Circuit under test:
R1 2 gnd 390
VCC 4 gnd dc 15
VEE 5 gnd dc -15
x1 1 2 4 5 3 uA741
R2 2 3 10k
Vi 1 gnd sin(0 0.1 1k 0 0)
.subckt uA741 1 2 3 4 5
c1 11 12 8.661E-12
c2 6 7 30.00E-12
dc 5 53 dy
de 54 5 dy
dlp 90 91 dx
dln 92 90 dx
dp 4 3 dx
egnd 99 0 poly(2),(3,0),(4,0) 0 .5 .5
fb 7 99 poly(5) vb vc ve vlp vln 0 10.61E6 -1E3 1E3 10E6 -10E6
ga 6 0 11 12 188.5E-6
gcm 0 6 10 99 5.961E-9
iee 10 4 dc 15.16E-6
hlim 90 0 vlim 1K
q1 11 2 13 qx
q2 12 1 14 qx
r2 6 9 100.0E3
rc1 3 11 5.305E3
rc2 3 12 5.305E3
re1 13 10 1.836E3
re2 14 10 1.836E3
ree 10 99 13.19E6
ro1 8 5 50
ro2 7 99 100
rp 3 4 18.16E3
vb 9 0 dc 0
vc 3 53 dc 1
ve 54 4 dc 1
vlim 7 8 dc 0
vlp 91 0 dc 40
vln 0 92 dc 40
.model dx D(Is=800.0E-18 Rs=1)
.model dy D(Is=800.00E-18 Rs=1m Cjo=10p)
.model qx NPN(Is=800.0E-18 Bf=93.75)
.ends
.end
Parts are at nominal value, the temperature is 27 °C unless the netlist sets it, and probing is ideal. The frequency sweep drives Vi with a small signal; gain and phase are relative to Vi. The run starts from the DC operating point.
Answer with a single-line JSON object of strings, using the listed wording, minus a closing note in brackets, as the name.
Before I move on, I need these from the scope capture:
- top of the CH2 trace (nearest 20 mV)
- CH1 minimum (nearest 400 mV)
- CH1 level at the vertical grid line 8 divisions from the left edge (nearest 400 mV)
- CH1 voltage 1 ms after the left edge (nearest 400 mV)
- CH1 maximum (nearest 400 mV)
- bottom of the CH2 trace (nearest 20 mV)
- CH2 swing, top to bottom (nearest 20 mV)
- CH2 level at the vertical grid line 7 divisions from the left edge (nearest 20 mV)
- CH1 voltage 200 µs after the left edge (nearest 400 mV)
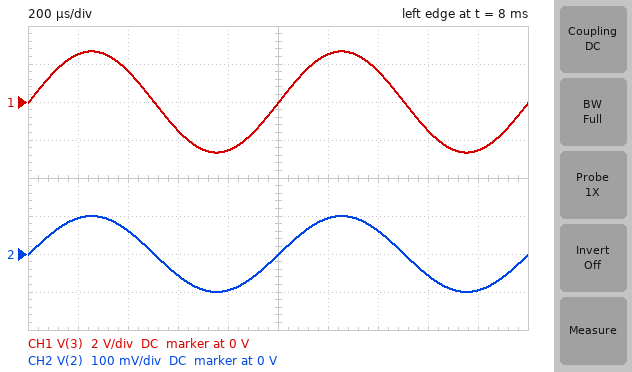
{"top of the CH2 trace": "100 mV", "CH1 minimum": "-2.8 V", "CH1 level at the vertical grid line 8 divisions from the left edge": "-1.6 V", "CH1 voltage 1 ms after the left edge": "0 V", "CH1 maximum": "2.8 V", "bottom of the CH2 trace": "-100 mV", "CH2 swing, top to bottom": "200 mV", "CH2 level at the vertical grid line 7 divisions from the left edge": "60 mV", "CH1 voltage 200 µs after the left edge": "2.4 V"}
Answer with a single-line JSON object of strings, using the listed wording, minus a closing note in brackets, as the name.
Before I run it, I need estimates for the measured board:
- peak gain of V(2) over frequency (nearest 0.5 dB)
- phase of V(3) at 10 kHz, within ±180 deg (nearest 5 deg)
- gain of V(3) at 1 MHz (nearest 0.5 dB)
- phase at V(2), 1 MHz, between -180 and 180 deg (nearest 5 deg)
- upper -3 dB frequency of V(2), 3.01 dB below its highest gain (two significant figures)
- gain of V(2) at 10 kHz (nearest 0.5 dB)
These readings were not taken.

{"peak gain of V(2) over frequency": "0 dB", "phase of V(3) at 10 kHz, within ±180 deg": "-15 deg", "gain of V(3) at 1 MHz": "-1.0 dB", "phase at V(2), 1 MHz, between -180 and 180 deg": "-120 deg", "upper -3 dB frequency of V(2), 3.01 dB below its highest gain": "38 kHz", "gain of V(2) at 10 kHz": "-0.5 dB"}
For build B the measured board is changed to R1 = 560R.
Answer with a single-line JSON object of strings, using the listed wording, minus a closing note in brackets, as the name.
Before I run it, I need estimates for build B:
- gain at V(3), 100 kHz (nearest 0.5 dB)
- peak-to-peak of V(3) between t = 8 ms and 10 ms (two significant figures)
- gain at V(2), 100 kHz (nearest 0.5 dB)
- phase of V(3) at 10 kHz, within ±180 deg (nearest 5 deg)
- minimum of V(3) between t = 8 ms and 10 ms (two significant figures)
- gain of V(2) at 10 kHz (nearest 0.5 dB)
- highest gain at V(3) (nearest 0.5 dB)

{"gain at V(3), 100 kHz": "19.0 dB", "peak-to-peak of V(3) between t = 8 ms and 10 ms": "3.8 V", "gain at V(2), 100 kHz": "-6.5 dB", "phase of V(3) at 10 kHz, within ±180 deg": "-10 deg", "minimum of V(3) between t = 8 ms and 10 ms": "-1.9 V", "gain of V(2) at 10 kHz": "0 dB", "highest gain at V(3)": "25.5 dB"}
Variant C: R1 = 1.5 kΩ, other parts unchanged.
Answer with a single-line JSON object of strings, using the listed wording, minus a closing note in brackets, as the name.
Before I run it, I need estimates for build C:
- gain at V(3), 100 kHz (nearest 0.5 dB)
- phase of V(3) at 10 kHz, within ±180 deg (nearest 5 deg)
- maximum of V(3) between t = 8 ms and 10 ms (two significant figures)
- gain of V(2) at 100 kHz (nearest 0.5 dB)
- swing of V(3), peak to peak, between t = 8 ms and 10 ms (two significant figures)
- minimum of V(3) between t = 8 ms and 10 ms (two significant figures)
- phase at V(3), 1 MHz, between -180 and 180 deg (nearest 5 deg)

{"gain at V(3), 100 kHz": "16.0 dB", "phase of V(3) at 10 kHz, within ±180 deg": "-5 deg", "maximum of V(3) between t = 8 ms and 10 ms": "770 mV", "gain of V(2) at 100 kHz": "-2.0 dB", "swing of V(3), peak to peak, between t = 8 ms and 10 ms": "1.5 V", "minimum of V(3) between t = 8 ms and 10 ms": "-770 mV", "phase at V(3), 1 MHz, between -180 and 180 deg": "-115 deg"}
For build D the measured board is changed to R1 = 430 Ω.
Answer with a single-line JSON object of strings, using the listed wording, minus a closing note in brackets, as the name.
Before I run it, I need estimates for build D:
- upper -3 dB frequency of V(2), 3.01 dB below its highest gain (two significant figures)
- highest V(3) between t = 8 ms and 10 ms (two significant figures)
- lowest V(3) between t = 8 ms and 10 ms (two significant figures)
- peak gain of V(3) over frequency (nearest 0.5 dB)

{"upper -3 dB frequency of V(2), 3.01 dB below its highest gain": "42 kHz", "highest V(3) between t = 8 ms and 10 ms": "2.4 V", "lowest V(3) between t = 8 ms and 10 ms": "-2.4 V", "peak gain of V(3) over frequency": "27.5 dB"}
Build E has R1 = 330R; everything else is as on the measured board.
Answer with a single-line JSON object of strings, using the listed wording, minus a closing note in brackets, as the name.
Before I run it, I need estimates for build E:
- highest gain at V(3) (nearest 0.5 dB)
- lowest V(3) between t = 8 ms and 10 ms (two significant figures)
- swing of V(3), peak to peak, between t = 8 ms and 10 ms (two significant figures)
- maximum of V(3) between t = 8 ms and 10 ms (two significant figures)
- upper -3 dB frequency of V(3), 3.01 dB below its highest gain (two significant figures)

{"highest gain at V(3)": "30.0 dB", "lowest V(3) between t = 8 ms and 10 ms": "-3.1 V", "swing of V(3), peak to peak, between t = 8 ms and 10 ms": "6.3 V", "maximum of V(3) between t = 8 ms and 10 ms": "3.1 V", "upper -3 dB frequency of V(3), 3.01 dB below its highest gain": "32 kHz"}
